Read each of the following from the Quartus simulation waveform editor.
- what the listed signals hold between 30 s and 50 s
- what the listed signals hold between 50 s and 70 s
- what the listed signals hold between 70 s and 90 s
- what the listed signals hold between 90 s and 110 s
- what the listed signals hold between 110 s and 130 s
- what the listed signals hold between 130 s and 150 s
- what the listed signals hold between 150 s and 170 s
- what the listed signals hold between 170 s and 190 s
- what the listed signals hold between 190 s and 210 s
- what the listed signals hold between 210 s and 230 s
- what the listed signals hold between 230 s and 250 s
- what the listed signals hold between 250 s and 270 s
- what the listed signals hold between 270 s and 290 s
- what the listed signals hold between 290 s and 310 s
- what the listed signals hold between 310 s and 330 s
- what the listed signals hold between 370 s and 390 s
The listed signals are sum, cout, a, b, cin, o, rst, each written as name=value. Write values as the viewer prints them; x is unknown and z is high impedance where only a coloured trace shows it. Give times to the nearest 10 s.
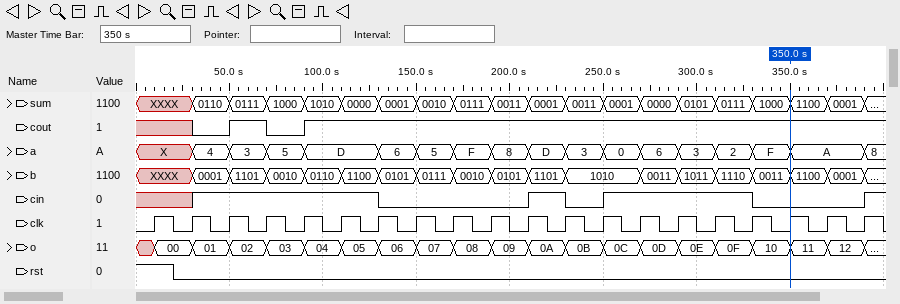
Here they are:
sum=0110, cout=0, a=4, b=0001, cin=1, o=01, rst=0
sum=0111, cout=1, a=3, b=1101, cin=1, o=02, rst=0
sum=1000, cout=0, a=5, b=0010, cin=1, o=03, rst=0
sum=1010, cout=1, a=D, b=0110, cin=1, o=04, rst=0
sum=0000, cout=1, a=D, b=1100, cin=1, o=05, rst=0
sum=0001, cout=1, a=6, b=0101, cin=0, o=06, rst=0
sum=0010, cout=1, a=5, b=0111, cin=0, o=07, rst=0
sum=0111, cout=1, a=F, b=0010, cin=0, o=08, rst=0
sum=0011, cout=1, a=8, b=0101, cin=0, o=09, rst=0
sum=0001, cout=1, a=D, b=1101, cin=1, o=0A, rst=0
sum=0011, cout=1, a=3, b=1010, cin=0, o=0B, rst=0
sum=0001, cout=1, a=0, b=1010, cin=1, o=0C, rst=0
sum=0000, cout=1, a=6, b=0011, cin=1, o=0D, rst=0
sum=0101, cout=1, a=3, b=1011, cin=1, o=0E, rst=0
sum=0111, cout=1, a=2, b=1110, cin=1, o=0F, rst=0
sum=0001, cout=1, a=A, b=0001, cin=0, o=12, rst=0
